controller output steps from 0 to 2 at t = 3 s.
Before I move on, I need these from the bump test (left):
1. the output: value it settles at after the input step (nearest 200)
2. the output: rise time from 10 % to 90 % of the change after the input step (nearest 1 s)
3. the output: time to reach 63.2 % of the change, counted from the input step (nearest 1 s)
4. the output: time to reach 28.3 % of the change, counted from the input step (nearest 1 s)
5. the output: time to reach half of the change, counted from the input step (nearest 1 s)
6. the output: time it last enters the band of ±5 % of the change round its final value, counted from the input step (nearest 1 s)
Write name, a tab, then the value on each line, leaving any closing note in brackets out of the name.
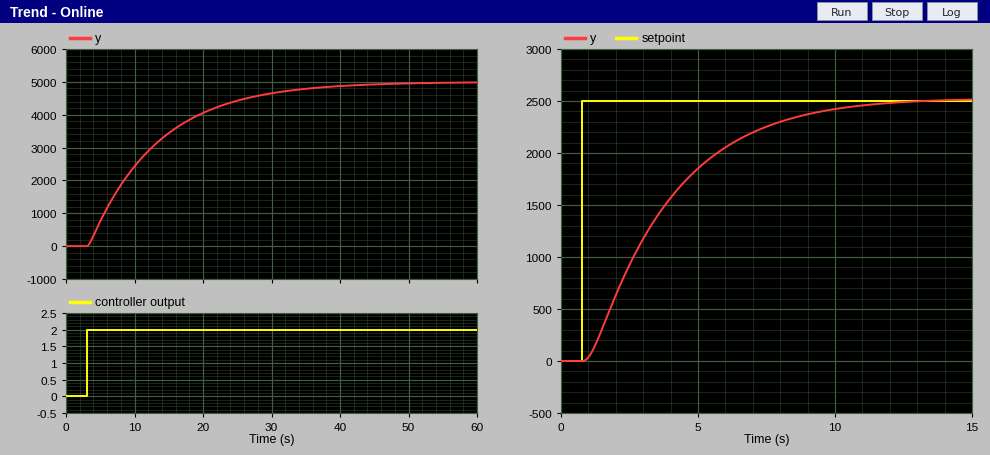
the output: value it settles at after the input step	5000
the output: rise time from 10 % to 90 % of the change after the input step	22 s
the output: time to reach 63.2 % of the change, counted from the input step	10 s
the output: time to reach 28.3 % of the change, counted from the input step	4 s
the output: time to reach half of the change, counted from the input step	7 s
the output: time it last enters the band of ±5 % of the change round its final value, counted from the input step	30 s
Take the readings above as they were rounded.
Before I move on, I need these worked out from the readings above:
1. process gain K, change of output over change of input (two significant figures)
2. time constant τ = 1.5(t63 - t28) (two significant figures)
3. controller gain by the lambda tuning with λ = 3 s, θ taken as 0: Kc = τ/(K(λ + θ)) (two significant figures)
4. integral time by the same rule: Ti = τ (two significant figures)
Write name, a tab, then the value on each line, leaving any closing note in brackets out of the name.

process gain K, change of output over change of input	2500
time constant τ = 1.5(t63 - t28)	9.0 s
controller gain by the lambda tuning with λ = 3 s, θ taken as 0: Kc = τ/(K(λ + θ))	0.0012
integral time by the same rule: Ti = τ	9.0 s
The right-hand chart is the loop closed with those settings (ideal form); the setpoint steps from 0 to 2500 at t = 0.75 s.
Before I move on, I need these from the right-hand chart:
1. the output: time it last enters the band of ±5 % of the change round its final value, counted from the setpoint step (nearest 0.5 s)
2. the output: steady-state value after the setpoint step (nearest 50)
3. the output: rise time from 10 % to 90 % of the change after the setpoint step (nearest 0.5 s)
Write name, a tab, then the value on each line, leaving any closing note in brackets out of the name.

the output: time it last enters the band of ±5 % of the change round its final value, counted from the setpoint step	8.5 s
the output: steady-state value after the setpoint step	2500
the output: rise time from 10 % to 90 % of the change after the setpoint step	6.0 s
